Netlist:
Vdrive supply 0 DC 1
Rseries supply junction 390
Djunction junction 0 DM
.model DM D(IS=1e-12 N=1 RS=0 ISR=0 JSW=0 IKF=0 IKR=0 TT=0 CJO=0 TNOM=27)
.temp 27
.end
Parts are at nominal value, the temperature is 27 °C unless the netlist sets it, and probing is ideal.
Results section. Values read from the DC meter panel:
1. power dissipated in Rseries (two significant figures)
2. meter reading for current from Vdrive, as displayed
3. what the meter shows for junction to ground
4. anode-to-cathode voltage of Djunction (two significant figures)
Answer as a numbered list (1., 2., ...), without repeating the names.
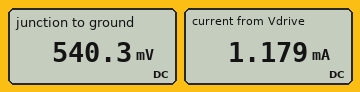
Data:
1. 540 µW
2. 1.179 mA
3. 540.3 mV
4. 540 mV
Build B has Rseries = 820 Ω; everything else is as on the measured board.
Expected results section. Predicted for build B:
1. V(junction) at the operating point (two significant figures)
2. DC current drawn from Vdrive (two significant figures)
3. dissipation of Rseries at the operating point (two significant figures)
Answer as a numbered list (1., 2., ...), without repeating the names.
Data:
1. 520 mV
2. 580 µA
3. 280 µW
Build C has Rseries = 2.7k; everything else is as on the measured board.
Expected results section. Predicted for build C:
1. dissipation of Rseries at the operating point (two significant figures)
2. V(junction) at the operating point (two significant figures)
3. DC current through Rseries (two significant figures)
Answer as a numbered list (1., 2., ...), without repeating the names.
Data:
1. 95 µW
2. 490 mV
3. 190 µA
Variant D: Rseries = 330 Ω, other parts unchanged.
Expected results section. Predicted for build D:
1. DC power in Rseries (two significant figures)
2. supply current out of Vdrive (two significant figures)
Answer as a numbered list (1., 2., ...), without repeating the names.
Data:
1. 630 µW
2. 1.4 mA
